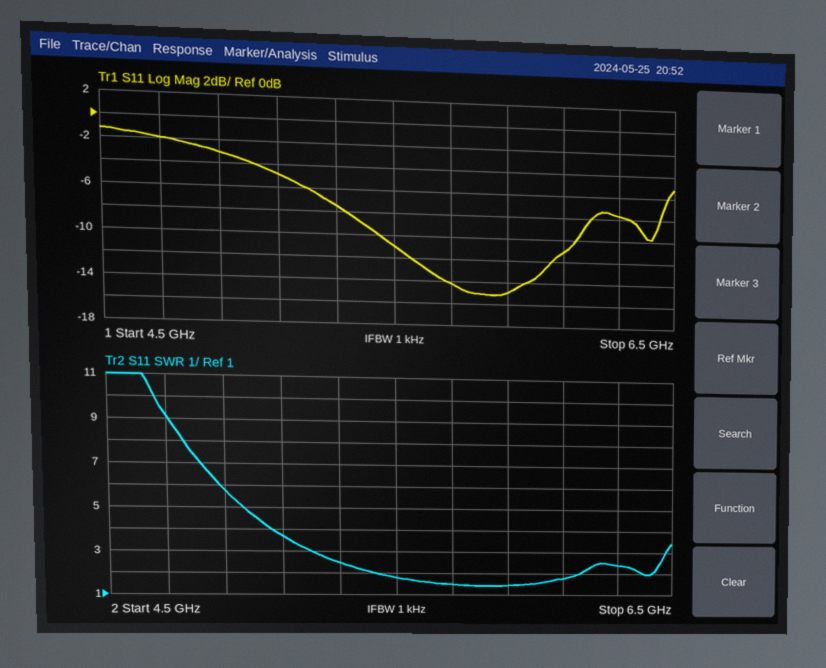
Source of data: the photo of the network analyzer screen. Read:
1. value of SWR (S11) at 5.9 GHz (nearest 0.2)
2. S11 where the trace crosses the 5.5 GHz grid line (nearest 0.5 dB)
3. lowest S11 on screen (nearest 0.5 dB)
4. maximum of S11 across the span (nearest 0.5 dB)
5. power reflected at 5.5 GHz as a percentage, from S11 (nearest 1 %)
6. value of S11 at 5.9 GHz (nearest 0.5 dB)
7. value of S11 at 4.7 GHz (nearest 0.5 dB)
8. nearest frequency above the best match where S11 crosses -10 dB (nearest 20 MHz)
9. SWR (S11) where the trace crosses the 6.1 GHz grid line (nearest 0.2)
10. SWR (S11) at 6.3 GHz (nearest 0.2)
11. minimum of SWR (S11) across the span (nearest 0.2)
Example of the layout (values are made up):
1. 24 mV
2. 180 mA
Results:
1. 1.4
2. -11.0 dB
3. -15.0 dB
4. -1.0 dB
5. 8 %
6. -15.0 dB
7. -2.0 dB
8. 6.14 GHz
9. 1.8
10. 2.4
11. 1.4
